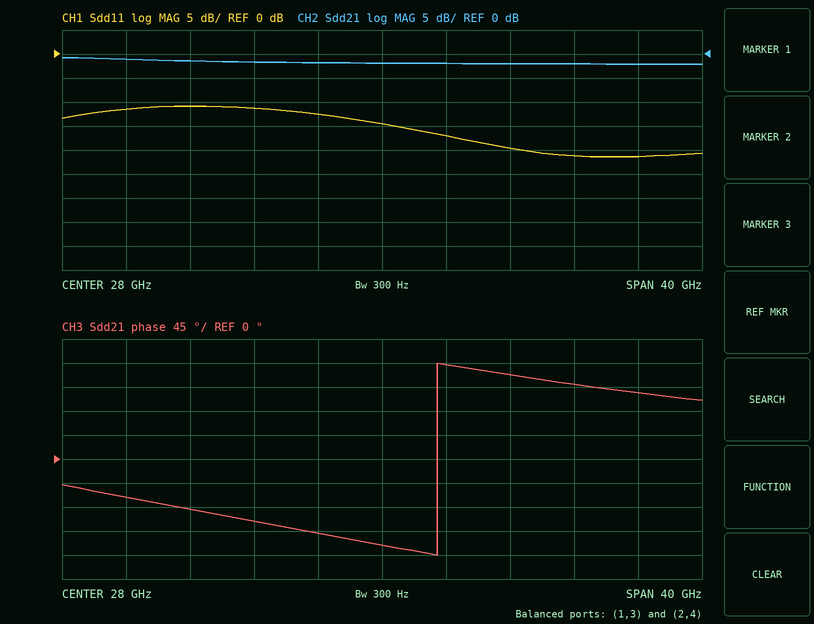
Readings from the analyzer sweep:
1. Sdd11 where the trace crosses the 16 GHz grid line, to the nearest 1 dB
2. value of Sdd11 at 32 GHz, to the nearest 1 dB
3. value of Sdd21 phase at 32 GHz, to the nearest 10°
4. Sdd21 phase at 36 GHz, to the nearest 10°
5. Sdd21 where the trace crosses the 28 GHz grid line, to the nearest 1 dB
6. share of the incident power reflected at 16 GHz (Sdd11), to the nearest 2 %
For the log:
-11 dB
-17 dB
180°
160°
-2 dB
8 %
